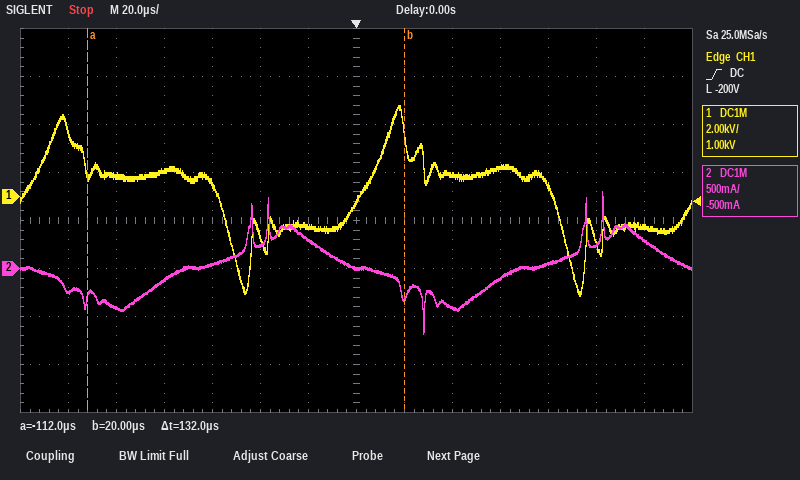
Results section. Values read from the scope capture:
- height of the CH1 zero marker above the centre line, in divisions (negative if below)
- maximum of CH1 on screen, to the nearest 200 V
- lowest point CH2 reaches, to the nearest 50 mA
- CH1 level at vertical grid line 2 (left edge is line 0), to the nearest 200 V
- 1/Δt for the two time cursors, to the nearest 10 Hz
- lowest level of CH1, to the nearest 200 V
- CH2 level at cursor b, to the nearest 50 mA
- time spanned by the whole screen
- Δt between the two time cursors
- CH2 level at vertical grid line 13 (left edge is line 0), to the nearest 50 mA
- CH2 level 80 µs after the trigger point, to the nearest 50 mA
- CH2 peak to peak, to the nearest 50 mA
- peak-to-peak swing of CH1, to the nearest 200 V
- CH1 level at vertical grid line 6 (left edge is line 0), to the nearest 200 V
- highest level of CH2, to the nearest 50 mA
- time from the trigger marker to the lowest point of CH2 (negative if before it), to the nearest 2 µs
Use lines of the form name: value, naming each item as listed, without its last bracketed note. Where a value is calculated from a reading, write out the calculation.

height of the CH1 zero marker above the centre line, in divisions: +0.5 div
maximum of CH1 on screen, to the nearest 200 V: 3.8 kV
lowest point CH2 reaches, to the nearest 50 mA: -700 mA
CH1 level at vertical grid line 2 (left edge is line 0), to the nearest 200 V: 800 V
1/Δt for the two time cursors, to the nearest 10 Hz: 1 / 132 µs ≈ 7.58 kHz
lowest level of CH1, to the nearest 200 V: -4.2 kV
CH2 level at cursor b, to the nearest 50 mA: -300 mA
time spanned by the whole screen: 280 µs
Δt between the two time cursors: 132 µs
CH2 level at vertical grid line 13 (left edge is line 0), to the nearest 50 mA: 300 mA
CH2 level 80 µs after the trigger point, to the nearest 50 mA: 50 mA
CH2 peak to peak, to the nearest 50 mA: 800 mA − (-700 mA) = 1.50 A
peak-to-peak swing of CH1, to the nearest 200 V: 3.8 kV − (-4.2 kV) = 8.0 kV
CH1 level at vertical grid line 6 (left edge is line 0), to the nearest 200 V: -1.2 kV
highest level of CH2, to the nearest 50 mA: 800 mA
time from the trigger marker to the lowest point of CH2 (negative if before it), to the nearest 2 µs: +28 µs
